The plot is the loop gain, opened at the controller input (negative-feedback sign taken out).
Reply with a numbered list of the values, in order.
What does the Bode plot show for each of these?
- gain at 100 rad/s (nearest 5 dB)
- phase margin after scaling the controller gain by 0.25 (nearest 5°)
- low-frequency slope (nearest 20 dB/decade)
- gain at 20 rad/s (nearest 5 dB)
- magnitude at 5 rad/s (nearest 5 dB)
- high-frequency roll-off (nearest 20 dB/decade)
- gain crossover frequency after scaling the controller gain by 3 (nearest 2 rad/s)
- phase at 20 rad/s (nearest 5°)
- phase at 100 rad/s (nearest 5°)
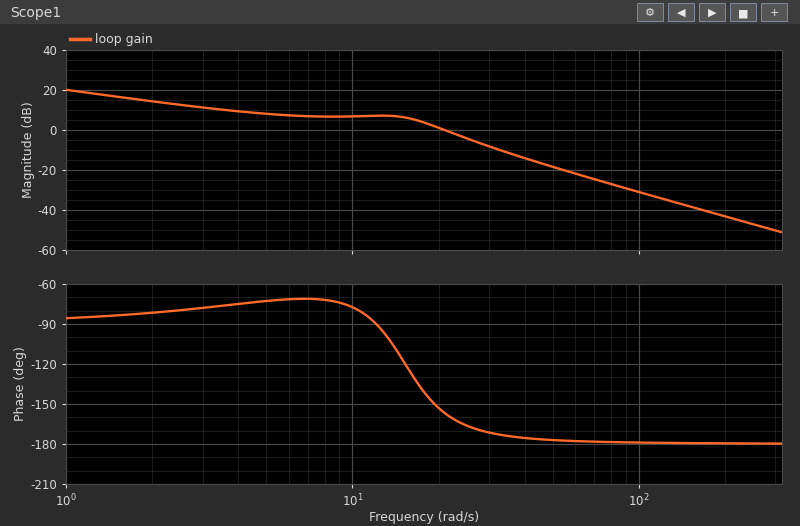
1. -30 dB
2. 100°
3. -20 dB/decade
4. 0 dB
5. 10 dB
6. -40 dB/decade
7. 32 rad/s
8. -155°
9. -180°
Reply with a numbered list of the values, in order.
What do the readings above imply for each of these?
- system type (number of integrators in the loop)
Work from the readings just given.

1. 1
